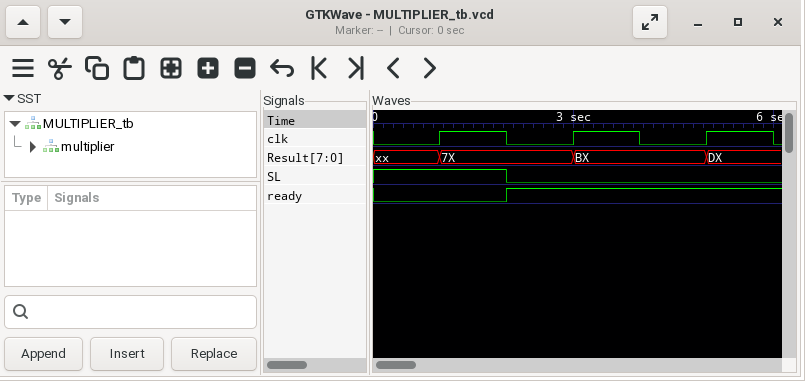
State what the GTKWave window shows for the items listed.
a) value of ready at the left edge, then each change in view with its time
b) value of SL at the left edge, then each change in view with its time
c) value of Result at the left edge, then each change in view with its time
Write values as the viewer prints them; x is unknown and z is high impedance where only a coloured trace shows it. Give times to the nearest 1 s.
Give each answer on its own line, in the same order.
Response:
0, 1 at 2 s
1, 0 at 2 s
xx, 7X at 1 s, BX at 3 s, DX at 5 s
